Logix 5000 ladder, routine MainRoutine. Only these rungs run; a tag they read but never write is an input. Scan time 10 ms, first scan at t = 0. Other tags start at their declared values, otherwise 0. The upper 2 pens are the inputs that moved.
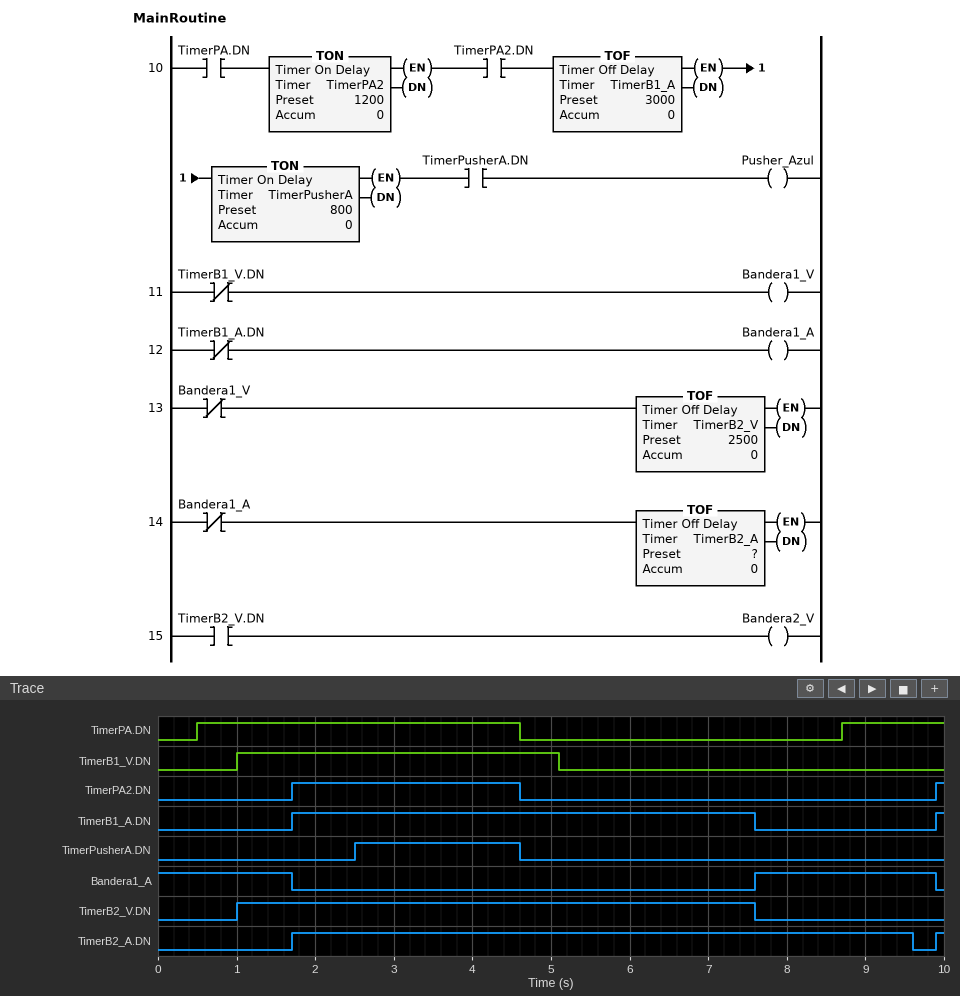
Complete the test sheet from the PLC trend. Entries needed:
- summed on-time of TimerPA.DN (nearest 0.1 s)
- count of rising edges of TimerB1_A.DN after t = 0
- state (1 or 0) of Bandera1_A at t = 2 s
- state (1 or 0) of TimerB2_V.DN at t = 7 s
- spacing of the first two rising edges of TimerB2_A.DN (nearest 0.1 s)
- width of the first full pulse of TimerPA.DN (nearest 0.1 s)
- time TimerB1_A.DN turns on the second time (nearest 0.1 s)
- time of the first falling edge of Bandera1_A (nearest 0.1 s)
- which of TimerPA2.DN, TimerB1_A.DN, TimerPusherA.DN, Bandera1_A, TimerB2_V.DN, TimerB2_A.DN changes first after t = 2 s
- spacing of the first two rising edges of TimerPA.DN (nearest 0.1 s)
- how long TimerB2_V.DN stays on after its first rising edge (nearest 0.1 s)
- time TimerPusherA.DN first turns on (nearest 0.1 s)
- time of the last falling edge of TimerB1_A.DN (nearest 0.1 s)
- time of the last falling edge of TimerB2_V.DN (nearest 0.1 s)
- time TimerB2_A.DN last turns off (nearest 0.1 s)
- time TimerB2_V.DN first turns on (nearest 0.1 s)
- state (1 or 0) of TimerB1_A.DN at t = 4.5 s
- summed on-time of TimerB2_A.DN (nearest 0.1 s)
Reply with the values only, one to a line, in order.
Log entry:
5.4 s
2
0
1
8.2 s
4.1 s
9.9 s
1.7 s
TimerPusherA.DN
8.2 s
6.6 s
2.5 s
7.6 s
7.6 s
9.6 s
1.0 s
1
8.0 s
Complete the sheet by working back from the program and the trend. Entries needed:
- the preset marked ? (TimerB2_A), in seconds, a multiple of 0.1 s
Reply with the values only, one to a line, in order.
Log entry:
2.0 s
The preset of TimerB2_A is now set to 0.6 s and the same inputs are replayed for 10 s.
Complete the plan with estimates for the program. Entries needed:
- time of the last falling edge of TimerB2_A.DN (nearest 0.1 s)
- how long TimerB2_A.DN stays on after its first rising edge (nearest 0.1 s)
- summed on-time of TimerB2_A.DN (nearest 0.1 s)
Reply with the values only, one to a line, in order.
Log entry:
8.2 s
6.5 s
6.6 s
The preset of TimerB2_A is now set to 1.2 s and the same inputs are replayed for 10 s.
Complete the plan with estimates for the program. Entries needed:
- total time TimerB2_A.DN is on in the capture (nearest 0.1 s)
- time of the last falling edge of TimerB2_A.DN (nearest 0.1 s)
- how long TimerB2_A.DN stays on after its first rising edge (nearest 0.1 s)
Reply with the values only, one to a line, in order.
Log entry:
7.2 s
8.8 s
7.1 s
